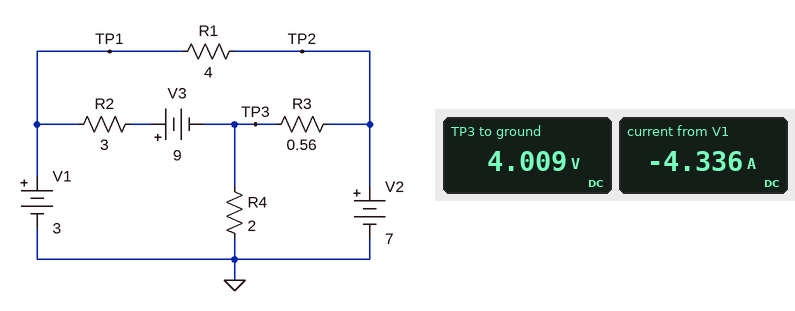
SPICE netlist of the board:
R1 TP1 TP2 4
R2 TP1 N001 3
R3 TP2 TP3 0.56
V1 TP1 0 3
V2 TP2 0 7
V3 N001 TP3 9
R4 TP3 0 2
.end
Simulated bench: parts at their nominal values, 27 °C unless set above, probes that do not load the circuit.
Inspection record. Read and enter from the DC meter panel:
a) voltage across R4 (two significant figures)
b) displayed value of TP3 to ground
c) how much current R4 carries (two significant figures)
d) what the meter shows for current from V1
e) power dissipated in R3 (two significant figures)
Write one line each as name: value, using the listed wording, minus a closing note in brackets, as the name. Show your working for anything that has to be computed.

voltage across R4: 4.009 V = 4.0 V
displayed value of TP3 to ground: 4.009 V
how much current R4 carries: (4.009 V) / 2 Ω = 2.0 A
what the meter shows for current from V1: -4.336 A
power dissipated in R3: (7 V - 4.009 V)^2 / 560 mΩ = 16 W
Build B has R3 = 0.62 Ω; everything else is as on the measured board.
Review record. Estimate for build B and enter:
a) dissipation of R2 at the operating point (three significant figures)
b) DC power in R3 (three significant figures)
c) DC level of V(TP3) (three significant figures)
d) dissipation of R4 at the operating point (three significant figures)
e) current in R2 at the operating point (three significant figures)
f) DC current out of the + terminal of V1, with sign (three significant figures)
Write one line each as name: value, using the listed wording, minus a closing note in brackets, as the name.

dissipation of R2 at the operating point: 32.0 W
DC power in R3: 16.5 W
DC level of V(TP3): 3.80 V
dissipation of R4 at the operating point: 7.21 W
current in R2 at the operating point: 3.27 A
DC current out of the + terminal of V1, with sign: -4.27 A
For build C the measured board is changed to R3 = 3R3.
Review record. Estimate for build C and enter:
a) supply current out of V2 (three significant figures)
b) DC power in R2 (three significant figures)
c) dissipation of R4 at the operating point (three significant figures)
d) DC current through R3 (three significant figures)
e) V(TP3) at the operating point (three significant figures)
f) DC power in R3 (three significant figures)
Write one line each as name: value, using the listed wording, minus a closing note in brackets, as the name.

supply current out of V2: 3.09 A
DC power in R2: 12.4 W
dissipation of R4 at the operating point: 5.69 mW
DC current through R3: 2.09 A
V(TP3) at the operating point: 107 mV
DC power in R3: 14.4 W
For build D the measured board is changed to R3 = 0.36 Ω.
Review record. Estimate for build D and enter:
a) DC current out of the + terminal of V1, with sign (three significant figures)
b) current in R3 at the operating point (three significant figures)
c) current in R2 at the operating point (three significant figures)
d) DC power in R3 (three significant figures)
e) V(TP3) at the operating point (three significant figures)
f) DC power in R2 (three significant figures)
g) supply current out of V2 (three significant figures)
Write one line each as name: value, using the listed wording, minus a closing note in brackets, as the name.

DC current out of the + terminal of V1, with sign: -4.61 A
current in R3 at the operating point: 6.03 A
current in R2 at the operating point: 3.61 A
DC power in R3: 13.1 W
V(TP3) at the operating point: 4.83 V
DC power in R2: 39.1 W
supply current out of V2: 7.03 A
